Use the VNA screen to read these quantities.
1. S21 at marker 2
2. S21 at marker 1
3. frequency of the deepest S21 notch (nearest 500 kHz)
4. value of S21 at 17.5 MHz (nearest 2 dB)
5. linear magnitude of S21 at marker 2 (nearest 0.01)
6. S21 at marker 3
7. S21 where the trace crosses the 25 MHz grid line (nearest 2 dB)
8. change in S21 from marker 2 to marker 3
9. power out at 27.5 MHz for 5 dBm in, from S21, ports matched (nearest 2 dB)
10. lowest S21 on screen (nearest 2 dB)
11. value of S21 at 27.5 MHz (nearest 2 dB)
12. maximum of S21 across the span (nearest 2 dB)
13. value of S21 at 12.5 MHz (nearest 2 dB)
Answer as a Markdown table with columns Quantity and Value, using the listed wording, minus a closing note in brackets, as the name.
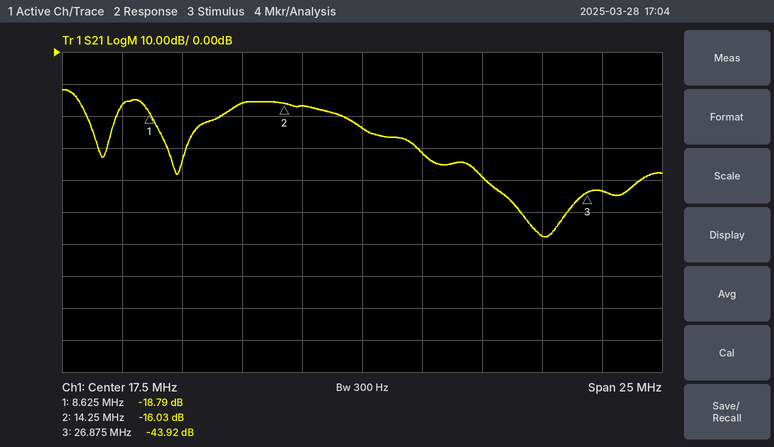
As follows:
| Quantity | Value |
|---|---|
| S21 at marker 2 | -16.03 dB |
| S21 at marker 1 | -18.79 dB |
| frequency of the deepest S21 notch | 25.0 MHz |
| value of S21 at 17.5 MHz | -24 dB |
| linear magnitude of S21 at marker 2 | 0.16 |
| S21 at marker 3 | -43.92 dB |
| S21 where the trace crosses the 25 MHz grid line | -58 dB |
| change in S21 from marker 2 to marker 3 | -27.89 dB |
| power out at 27.5 MHz for 5 dBm in, from S21, ports matched | -38 dBm |
| lowest S21 on screen | -58 dB |
| value of S21 at 27.5 MHz | -44 dB |
| maximum of S21 across the span | -12 dB |
| value of S21 at 12.5 MHz | -16 dB |
